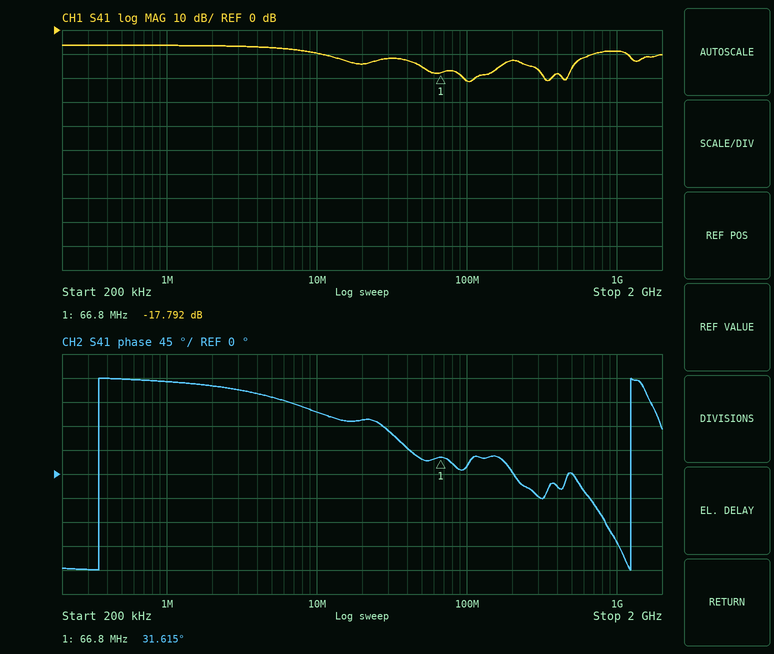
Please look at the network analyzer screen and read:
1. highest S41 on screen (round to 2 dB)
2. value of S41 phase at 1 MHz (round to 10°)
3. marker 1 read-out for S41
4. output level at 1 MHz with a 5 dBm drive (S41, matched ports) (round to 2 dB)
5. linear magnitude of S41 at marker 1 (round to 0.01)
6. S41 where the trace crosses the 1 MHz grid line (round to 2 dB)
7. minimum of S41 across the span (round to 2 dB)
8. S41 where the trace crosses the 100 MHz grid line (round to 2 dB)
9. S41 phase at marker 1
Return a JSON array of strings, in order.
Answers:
["-6 dB", "170°", "-17.792 dB", "-2 dBm", "0.13", "-6 dB", "-22 dB", "-22 dB", "31.615°"]
